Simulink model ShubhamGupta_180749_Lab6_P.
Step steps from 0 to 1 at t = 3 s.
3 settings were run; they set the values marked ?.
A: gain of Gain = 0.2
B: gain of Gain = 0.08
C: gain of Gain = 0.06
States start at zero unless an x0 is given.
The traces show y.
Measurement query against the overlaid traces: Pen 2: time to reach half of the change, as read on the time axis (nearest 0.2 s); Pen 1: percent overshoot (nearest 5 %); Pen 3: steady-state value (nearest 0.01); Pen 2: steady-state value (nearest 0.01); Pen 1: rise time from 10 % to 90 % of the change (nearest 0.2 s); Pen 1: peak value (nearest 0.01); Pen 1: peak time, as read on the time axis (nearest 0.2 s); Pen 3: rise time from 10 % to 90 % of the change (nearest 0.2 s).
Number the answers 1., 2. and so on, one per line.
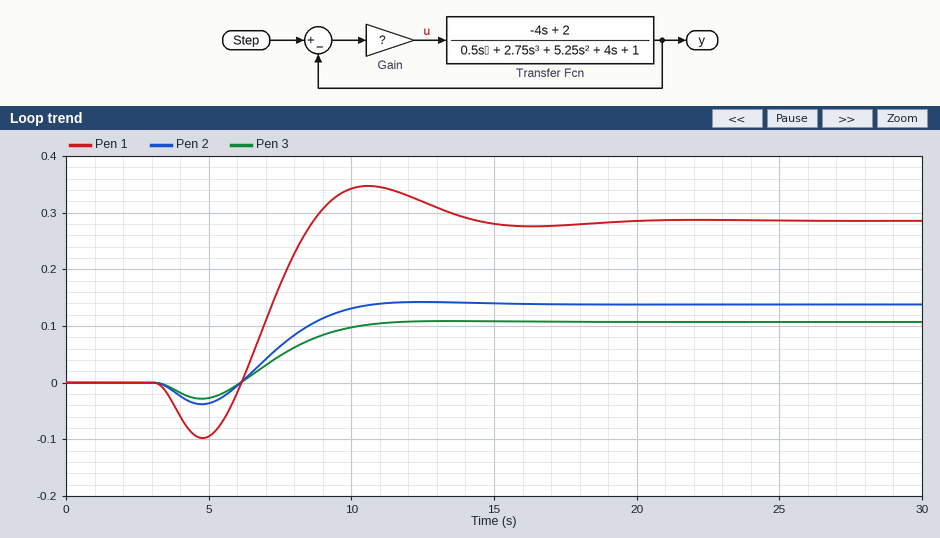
1. 7.6 s
2. 20 %
3. 0.11
4. 0.14
5. 2.0 s
6. 0.35
7. 10.6 s
8. 3.4 s
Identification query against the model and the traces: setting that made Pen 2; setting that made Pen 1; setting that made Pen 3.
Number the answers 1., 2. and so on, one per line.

1. B
2. A
3. C
